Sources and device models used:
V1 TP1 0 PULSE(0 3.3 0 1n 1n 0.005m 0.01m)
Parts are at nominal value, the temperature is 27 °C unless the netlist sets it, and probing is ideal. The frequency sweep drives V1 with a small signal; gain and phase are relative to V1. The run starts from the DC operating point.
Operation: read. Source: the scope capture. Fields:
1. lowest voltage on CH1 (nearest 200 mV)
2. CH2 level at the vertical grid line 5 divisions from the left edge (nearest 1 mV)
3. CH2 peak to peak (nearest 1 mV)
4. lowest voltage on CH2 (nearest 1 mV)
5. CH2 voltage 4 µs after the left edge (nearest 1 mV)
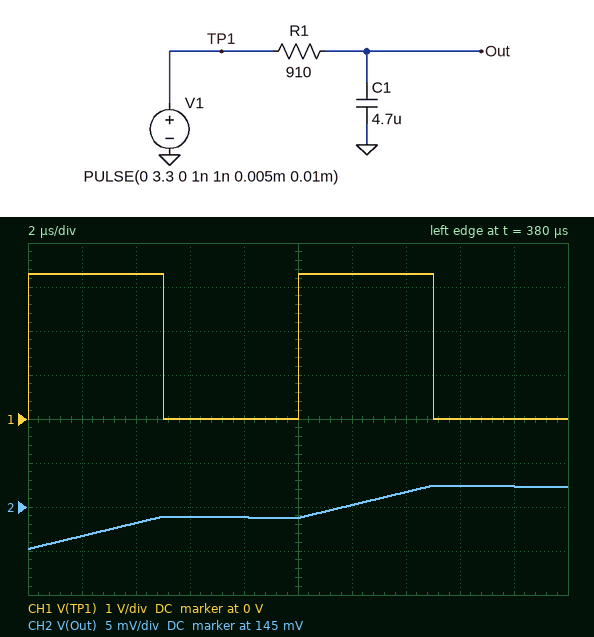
0 V
144 mV
7 mV
140 mV
143 mV
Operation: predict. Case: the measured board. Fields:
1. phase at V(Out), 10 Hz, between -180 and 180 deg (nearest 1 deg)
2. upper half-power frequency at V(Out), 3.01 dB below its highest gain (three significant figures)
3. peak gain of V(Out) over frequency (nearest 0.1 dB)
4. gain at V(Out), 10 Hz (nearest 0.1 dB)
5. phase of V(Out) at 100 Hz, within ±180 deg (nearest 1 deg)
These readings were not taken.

-15 deg
37.2 Hz
0 dB
-0.3 dB
-70 deg
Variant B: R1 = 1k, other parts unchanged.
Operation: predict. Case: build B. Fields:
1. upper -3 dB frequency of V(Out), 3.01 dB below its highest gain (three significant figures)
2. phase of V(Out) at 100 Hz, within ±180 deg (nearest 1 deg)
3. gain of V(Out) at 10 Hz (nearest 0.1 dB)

33.9 Hz
-71 deg
-0.4 dB
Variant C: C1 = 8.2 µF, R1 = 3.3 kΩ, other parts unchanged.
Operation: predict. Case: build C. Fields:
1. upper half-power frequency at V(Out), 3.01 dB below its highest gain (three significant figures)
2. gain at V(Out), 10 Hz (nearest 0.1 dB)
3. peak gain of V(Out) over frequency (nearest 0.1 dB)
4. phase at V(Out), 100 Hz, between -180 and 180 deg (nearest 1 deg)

5.88 Hz
-5.9 dB
0 dB
-87 deg
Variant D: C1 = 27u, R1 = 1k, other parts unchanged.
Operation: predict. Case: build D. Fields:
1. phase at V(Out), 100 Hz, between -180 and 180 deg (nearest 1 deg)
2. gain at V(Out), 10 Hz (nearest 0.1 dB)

-87 deg
-5.9 dB
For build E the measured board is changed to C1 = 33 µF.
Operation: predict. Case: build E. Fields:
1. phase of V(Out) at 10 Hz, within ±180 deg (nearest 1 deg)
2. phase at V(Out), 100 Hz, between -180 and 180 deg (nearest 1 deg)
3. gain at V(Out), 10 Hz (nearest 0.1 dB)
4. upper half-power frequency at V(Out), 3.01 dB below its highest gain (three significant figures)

-62 deg
-87 deg
-6.6 dB
5.30 Hz
